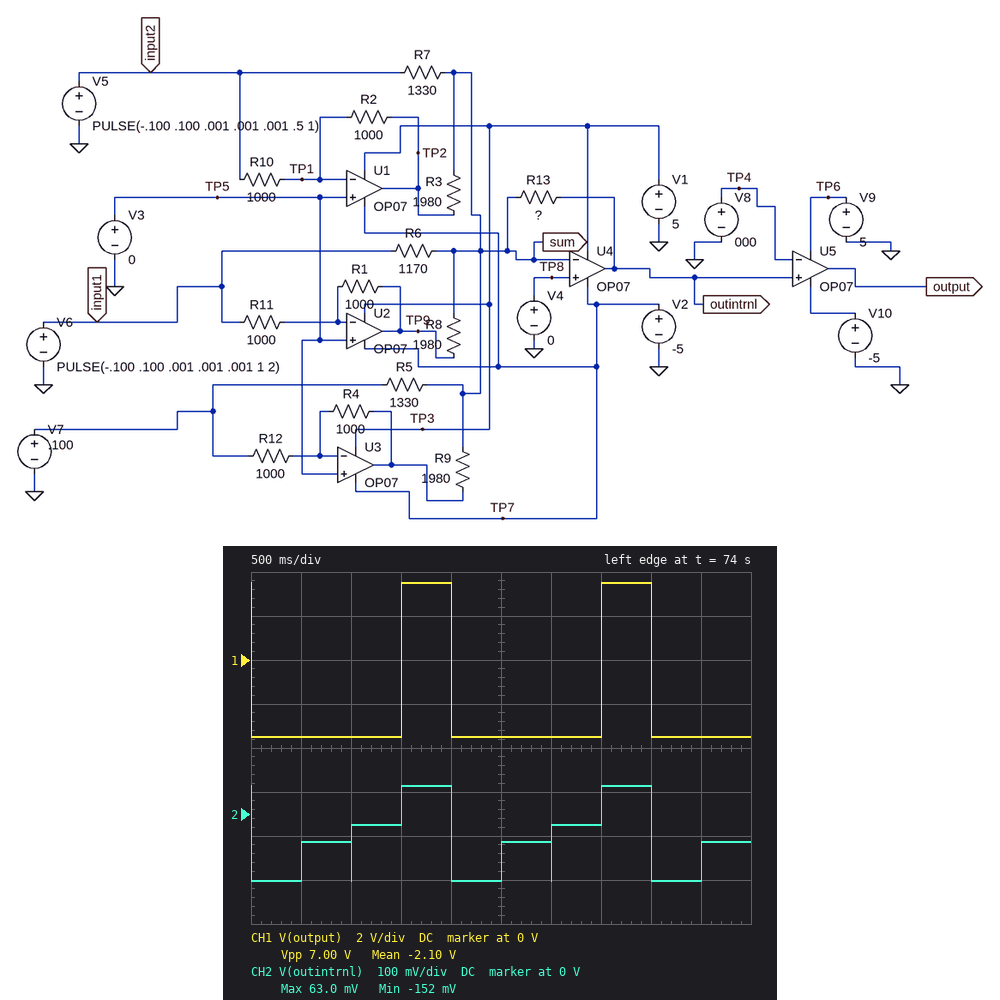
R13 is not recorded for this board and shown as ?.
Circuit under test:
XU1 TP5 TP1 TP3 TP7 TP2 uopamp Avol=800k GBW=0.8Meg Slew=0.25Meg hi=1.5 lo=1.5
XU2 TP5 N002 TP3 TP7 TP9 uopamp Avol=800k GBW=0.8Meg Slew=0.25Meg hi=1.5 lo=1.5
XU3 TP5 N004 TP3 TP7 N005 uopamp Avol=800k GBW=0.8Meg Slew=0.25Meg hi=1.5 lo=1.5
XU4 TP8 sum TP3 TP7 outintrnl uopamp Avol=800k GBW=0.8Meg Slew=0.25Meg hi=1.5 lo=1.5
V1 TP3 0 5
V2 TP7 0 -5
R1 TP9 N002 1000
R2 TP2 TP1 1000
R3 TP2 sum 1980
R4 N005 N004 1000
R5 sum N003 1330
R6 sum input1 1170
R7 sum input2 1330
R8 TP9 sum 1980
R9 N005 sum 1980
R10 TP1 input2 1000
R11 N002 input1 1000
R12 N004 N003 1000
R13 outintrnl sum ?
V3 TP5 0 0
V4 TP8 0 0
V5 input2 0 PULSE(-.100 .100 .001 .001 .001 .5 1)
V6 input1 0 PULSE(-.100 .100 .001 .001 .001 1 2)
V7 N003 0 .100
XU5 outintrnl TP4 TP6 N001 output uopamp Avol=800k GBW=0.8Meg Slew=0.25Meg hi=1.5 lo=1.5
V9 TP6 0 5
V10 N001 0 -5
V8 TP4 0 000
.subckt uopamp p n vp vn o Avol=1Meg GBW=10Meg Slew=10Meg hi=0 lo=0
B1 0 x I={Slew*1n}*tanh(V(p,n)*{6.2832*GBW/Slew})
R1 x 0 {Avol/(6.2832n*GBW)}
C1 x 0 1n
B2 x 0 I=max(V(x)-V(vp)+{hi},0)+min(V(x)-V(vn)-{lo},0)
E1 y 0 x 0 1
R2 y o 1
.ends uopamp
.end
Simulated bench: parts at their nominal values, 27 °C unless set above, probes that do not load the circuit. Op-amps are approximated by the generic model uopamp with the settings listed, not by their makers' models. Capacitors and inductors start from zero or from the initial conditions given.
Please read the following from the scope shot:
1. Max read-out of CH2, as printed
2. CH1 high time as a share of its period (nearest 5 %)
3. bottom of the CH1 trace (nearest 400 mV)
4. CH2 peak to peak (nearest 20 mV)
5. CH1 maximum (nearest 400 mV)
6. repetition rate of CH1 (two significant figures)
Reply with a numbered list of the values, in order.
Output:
1. 63.0 mV
2. 25 %
3. -3.6 V
4. 220 mV
5. 3.6 V
6. 500 mHz
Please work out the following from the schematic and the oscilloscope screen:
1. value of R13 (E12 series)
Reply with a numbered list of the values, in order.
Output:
1. 1.8 kΩ
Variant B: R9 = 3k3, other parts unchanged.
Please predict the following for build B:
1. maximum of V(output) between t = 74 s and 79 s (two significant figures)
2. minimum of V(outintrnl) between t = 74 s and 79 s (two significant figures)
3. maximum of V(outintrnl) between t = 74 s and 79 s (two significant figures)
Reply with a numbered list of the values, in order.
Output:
1. 3.5 V
2. -190 mV
3. 27 mV
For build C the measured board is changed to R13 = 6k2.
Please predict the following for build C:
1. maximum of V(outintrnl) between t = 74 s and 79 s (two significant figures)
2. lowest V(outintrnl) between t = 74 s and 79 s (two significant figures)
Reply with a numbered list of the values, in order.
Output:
1. 220 mV
2. -520 mV
